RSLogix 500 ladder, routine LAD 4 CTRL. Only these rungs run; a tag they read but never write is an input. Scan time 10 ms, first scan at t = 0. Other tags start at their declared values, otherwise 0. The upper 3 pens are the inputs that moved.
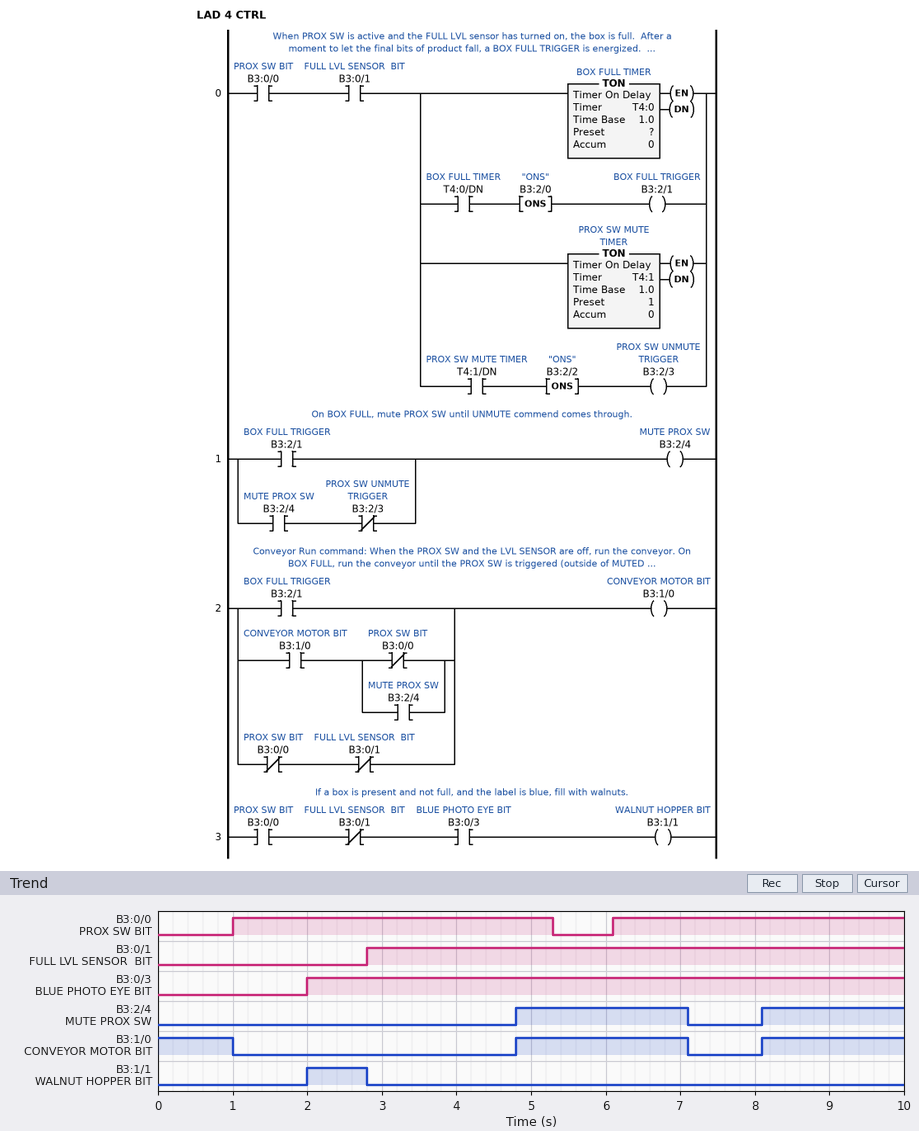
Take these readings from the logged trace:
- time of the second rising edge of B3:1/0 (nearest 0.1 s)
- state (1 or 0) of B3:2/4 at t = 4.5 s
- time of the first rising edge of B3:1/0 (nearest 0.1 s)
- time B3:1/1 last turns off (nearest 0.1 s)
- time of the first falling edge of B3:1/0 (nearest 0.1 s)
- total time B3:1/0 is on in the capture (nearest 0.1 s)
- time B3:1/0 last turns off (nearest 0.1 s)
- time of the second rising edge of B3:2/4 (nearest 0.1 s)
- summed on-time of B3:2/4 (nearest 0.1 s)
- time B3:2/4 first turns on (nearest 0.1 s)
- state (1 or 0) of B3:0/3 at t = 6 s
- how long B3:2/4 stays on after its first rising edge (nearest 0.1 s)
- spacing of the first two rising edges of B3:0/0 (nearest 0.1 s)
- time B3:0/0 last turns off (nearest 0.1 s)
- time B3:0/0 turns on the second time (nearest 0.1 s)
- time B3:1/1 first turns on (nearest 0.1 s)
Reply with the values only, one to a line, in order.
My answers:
8.1 s
0
4.8 s
2.8 s
1.0 s
5.2 s
7.1 s
8.1 s
4.2 s
4.8 s
1
2.3 s
5.1 s
5.3 s
6.1 s
2.0 s
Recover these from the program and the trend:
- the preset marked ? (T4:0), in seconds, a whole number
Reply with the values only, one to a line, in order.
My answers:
2 s
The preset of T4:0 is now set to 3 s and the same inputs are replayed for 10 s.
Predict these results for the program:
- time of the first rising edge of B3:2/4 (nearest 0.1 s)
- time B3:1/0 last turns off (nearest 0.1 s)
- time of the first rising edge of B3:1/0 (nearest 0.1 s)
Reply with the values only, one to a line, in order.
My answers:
9.1 s
1.0 s
9.1 s
